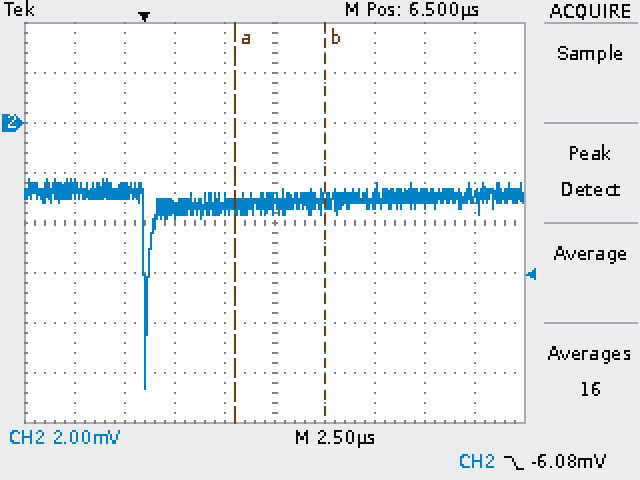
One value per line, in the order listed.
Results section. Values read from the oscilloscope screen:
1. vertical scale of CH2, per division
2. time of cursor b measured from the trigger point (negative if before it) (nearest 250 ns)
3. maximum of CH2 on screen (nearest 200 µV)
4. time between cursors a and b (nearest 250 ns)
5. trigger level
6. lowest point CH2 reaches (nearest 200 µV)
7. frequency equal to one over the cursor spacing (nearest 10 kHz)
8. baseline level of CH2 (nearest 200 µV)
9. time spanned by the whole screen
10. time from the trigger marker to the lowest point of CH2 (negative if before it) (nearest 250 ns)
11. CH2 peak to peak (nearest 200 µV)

2 mV
+9.00 µs
-2.2 mV
4.50 µs
-6.08 mV
-10.6 mV
220 kHz
-3.0 mV
25 µs
0.00 µs
8.4 mV
